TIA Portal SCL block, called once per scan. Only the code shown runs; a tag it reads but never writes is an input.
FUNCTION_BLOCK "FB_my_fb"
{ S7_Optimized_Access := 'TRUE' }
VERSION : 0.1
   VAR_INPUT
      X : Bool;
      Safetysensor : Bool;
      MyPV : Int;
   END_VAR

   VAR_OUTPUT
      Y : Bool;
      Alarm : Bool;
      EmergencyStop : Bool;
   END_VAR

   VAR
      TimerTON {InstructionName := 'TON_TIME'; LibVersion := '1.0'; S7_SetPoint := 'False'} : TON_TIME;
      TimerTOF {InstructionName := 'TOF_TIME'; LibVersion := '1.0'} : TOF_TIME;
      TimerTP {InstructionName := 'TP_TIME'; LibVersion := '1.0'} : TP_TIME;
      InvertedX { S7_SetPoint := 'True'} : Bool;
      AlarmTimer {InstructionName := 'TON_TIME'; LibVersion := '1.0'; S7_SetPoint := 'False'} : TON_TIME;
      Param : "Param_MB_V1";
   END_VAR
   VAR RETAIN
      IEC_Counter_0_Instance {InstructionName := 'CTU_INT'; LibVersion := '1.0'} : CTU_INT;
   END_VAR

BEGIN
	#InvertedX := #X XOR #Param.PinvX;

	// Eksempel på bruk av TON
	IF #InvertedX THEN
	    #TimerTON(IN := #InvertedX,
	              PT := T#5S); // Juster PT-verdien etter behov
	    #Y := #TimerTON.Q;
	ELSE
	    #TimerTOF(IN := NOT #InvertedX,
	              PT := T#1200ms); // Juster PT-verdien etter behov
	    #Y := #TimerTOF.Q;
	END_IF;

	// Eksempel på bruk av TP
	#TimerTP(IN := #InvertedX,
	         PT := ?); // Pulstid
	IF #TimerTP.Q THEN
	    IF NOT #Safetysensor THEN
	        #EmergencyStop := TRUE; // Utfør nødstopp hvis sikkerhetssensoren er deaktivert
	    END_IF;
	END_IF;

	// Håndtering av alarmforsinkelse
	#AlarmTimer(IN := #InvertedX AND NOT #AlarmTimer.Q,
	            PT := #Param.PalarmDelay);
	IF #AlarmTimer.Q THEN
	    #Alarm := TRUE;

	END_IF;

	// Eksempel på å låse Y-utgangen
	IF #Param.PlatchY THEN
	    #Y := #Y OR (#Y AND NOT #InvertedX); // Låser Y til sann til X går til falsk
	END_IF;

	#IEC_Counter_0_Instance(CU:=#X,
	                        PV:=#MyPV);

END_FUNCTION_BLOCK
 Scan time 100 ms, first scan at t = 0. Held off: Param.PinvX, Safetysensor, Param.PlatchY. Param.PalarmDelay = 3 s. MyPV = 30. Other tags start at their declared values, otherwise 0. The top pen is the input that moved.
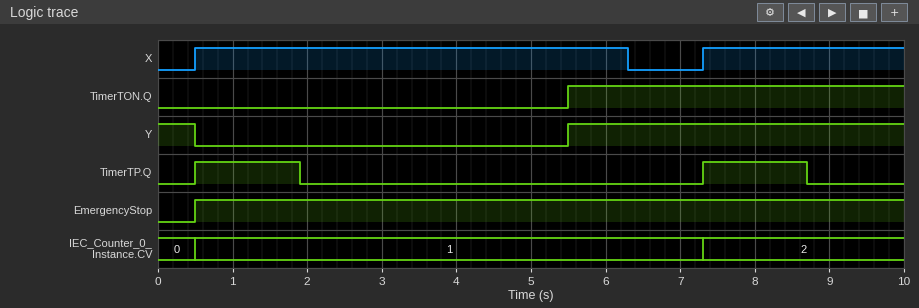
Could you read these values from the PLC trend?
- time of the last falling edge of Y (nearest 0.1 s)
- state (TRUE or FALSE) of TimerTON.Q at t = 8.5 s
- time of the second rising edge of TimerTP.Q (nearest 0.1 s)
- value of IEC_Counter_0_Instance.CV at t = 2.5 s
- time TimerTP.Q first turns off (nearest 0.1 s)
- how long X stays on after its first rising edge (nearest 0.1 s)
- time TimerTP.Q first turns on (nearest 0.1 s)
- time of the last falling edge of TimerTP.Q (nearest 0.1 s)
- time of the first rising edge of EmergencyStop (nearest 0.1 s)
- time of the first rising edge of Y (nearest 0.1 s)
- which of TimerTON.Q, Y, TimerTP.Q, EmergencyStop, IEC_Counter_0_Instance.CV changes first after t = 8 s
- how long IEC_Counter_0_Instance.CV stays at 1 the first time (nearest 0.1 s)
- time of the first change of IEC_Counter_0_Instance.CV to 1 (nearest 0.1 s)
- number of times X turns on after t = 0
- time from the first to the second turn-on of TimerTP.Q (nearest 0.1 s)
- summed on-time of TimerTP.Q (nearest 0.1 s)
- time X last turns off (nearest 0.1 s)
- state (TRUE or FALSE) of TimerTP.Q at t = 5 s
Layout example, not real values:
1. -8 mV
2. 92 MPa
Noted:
1. 0.5 s
2. TRUE
3. 7.3 s
4. 1
5. 1.9 s
6. 5.8 s
7. 0.5 s
8. 8.7 s
9. 0.5 s
10. 5.5 s
11. TimerTP.Q
12. 6.8 s
13. 0.5 s
14. 2
15. 6.8 s
16. 2.8 s
17. 6.3 s
18. FALSE
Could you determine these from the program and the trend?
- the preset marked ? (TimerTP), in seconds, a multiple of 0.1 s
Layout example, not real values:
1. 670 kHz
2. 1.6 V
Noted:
1. 1.4 s
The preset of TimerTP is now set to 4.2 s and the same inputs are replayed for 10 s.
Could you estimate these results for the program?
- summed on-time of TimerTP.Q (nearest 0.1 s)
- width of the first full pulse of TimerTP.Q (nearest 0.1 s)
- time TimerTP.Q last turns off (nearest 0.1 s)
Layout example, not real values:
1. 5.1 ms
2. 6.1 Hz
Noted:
1. 6.9 s
2. 4.2 s
3. 4.7 s
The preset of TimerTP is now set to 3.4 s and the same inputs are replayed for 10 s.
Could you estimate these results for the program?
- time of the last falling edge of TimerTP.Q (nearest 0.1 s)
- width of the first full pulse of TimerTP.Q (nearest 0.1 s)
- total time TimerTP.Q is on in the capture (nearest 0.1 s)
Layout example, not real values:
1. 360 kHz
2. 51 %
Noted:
1. 3.9 s
2. 3.4 s
3. 6.1 s
